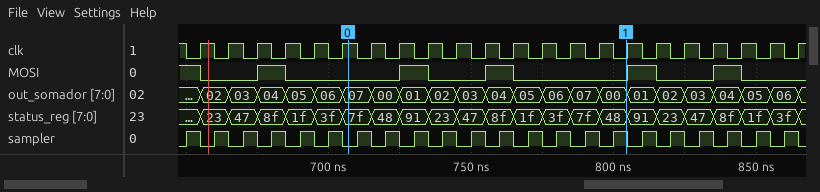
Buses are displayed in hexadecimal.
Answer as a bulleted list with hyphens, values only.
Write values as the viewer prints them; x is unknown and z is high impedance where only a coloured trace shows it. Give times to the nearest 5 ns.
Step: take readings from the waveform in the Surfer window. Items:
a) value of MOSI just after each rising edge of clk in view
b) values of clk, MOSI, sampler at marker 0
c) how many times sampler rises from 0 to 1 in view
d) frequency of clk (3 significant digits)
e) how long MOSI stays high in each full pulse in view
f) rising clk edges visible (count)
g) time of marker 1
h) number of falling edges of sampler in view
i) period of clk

- 0 0 1 0 0 0 0 1 0 0 1 0 0 0 0 1 0 0 1 0 0 0
- clk=1, MOSI=0, sampler=0
- 22
- 100 MHz
- 10 ns, 10 ns, 10 ns, 10 ns, 10 ns
- 22
- 805 ns
- 22
- 10 ns
